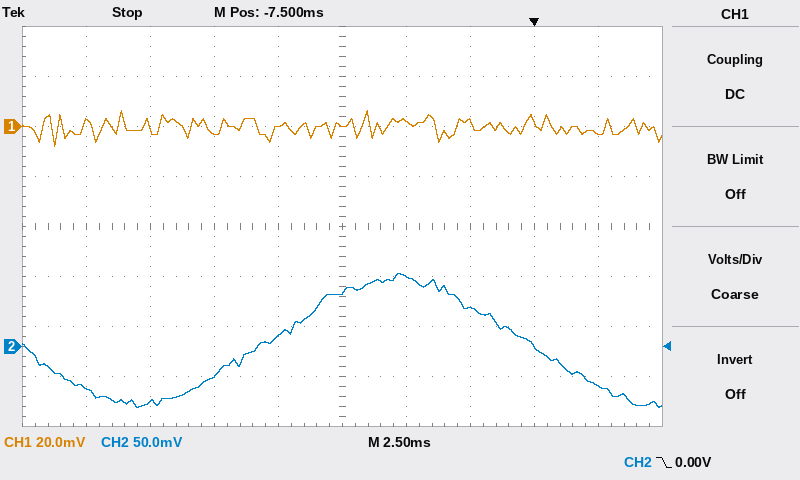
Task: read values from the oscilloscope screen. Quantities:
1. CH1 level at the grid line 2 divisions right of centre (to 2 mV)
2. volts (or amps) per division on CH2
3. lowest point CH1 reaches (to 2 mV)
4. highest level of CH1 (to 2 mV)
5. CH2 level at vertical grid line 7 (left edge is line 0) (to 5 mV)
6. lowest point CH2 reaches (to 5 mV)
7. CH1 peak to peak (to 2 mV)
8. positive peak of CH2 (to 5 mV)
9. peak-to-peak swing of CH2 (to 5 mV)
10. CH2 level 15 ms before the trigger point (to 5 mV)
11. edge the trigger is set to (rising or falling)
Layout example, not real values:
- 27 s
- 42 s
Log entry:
- 2 mV
- 50 mV
- -8 mV
- 6 mV
- 40 mV
- -60 mV
- 14 mV
- 75 mV
- 135 mV
- -55 mV
- falling
